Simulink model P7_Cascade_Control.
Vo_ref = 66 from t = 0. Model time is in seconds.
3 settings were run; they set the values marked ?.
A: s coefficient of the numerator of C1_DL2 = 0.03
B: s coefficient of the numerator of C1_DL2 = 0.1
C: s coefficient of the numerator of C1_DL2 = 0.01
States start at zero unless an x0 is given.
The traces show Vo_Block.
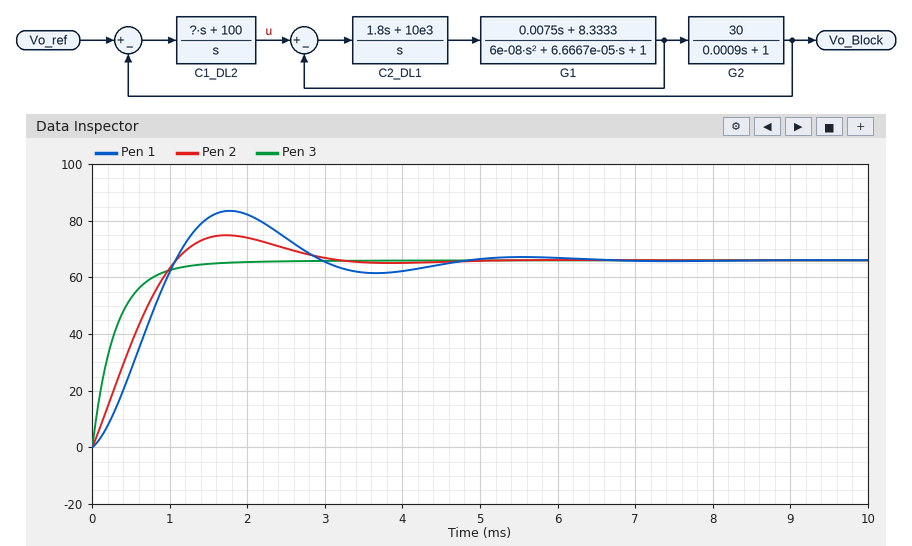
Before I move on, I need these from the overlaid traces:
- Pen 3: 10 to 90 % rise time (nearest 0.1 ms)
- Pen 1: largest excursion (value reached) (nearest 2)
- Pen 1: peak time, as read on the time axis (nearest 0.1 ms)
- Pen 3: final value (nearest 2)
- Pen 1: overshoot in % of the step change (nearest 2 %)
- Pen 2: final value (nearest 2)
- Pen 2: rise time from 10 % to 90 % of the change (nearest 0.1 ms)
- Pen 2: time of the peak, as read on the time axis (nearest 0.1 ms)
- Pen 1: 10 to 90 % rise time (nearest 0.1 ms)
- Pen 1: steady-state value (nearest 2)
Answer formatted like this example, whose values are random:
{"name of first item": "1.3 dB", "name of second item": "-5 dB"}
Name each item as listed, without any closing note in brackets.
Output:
{"Pen 3: 10 to 90 % rise time": "0.7 ms", "Pen 1: largest excursion (value reached)": "84", "Pen 1: peak time, as read on the time axis": "1.8 ms", "Pen 3: final value": "66", "Pen 1: overshoot in % of the step change": "26 %", "Pen 2: final value": "66", "Pen 2: rise time from 10 % to 90 % of the change": "0.8 ms", "Pen 2: time of the peak, as read on the time axis": "1.7 ms", "Pen 1: 10 to 90 % rise time": "0.8 ms", "Pen 1: steady-state value": "66"}
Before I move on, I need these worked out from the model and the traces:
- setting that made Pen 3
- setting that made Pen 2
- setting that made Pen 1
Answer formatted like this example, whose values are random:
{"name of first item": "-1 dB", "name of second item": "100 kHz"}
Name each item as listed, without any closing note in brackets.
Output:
{"setting that made Pen 3": "B", "setting that made Pen 2": "A", "setting that made Pen 1": "C"}
